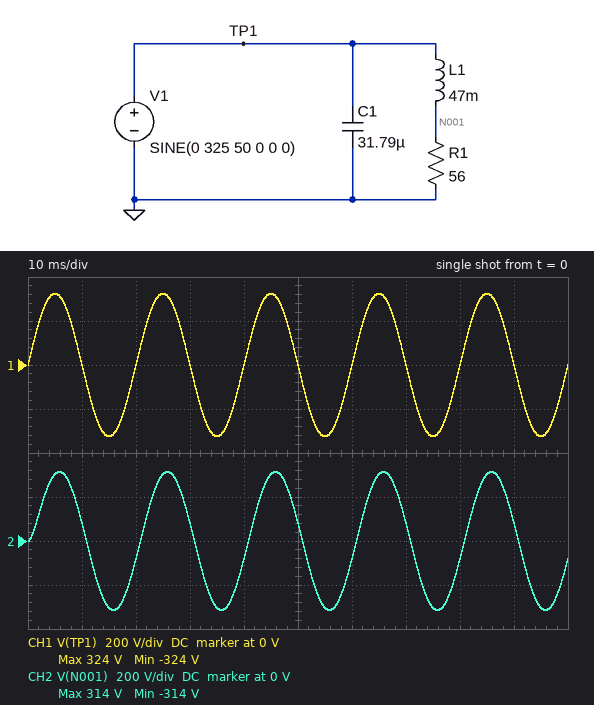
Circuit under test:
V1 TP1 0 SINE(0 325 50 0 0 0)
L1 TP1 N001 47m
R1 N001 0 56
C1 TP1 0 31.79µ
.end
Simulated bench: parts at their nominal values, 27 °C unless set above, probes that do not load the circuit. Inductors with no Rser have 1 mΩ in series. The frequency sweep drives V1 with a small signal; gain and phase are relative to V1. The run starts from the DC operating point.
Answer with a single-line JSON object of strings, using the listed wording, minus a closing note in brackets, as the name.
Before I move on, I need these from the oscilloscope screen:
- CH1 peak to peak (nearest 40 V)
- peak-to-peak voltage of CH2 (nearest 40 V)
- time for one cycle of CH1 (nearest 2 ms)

{"CH1 peak to peak": "640 V", "peak-to-peak voltage of CH2": "640 V", "time for one cycle of CH1": "20 ms"}
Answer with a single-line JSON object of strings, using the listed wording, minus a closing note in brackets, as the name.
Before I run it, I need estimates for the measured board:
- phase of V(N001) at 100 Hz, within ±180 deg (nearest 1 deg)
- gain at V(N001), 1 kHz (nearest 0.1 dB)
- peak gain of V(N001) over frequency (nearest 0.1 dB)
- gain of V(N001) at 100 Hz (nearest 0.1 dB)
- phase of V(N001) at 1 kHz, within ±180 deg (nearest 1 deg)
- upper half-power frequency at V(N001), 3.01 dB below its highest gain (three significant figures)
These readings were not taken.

{"phase of V(N001) at 100 Hz, within ±180 deg": "-28 deg", "gain at V(N001), 1 kHz": "-14.6 dB", "peak gain of V(N001) over frequency": "0 dB", "gain of V(N001) at 100 Hz": "-1.1 dB", "phase of V(N001) at 1 kHz, within ±180 deg": "-79 deg", "upper half-power frequency at V(N001), 3.01 dB below its highest gain": "190 Hz"}
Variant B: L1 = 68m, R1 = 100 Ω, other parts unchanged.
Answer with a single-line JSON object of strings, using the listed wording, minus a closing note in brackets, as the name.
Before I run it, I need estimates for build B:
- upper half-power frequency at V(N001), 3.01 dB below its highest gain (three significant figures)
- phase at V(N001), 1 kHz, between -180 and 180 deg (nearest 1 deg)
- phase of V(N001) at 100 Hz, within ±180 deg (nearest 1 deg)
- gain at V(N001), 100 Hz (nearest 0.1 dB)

{"upper half-power frequency at V(N001), 3.01 dB below its highest gain": "234 Hz", "phase at V(N001), 1 kHz, between -180 and 180 deg": "-77 deg", "phase of V(N001) at 100 Hz, within ±180 deg": "-23 deg", "gain at V(N001), 100 Hz": "-0.7 dB"}
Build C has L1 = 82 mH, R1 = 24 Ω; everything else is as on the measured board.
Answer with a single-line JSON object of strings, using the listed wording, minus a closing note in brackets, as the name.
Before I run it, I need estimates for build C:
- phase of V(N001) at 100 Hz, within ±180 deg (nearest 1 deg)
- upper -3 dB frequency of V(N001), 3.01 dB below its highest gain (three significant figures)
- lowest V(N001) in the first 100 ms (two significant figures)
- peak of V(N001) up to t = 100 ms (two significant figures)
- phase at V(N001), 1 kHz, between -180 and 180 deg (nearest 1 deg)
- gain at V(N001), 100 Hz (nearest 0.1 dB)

{"phase of V(N001) at 100 Hz, within ±180 deg": "-65 deg", "upper -3 dB frequency of V(N001), 3.01 dB below its highest gain": "46.6 Hz", "lowest V(N001) in the first 100 ms": "-220 V", "peak of V(N001) up to t = 100 ms": "240 V", "phase at V(N001), 1 kHz, between -180 and 180 deg": "-87 deg", "gain at V(N001), 100 Hz": "-7.5 dB"}
